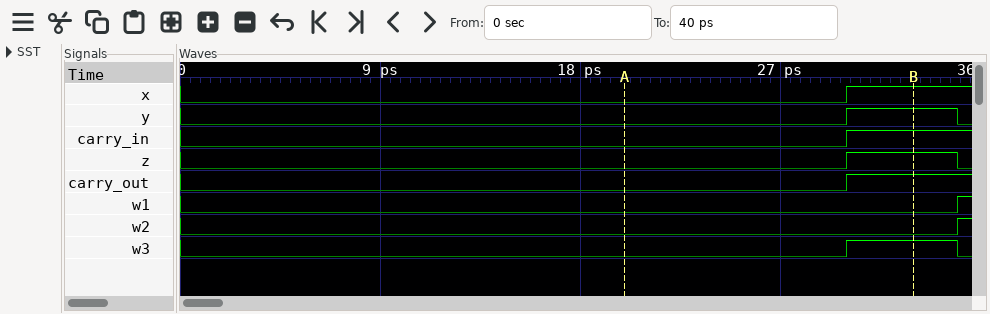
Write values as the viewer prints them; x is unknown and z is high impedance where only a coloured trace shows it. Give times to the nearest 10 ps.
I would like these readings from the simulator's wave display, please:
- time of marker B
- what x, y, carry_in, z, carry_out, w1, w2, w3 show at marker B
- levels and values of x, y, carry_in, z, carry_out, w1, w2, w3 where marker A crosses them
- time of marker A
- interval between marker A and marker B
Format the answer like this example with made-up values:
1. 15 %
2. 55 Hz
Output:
1. 30 ps
2. x=1, y=1, carry_in=1, z=1, carry_out=1, w1=0, w2=0, w3=1
3. x=0, y=0, carry_in=0, z=0, carry_out=0, w1=0, w2=0, w3=0
4. 20 ps
5. 10 ps
